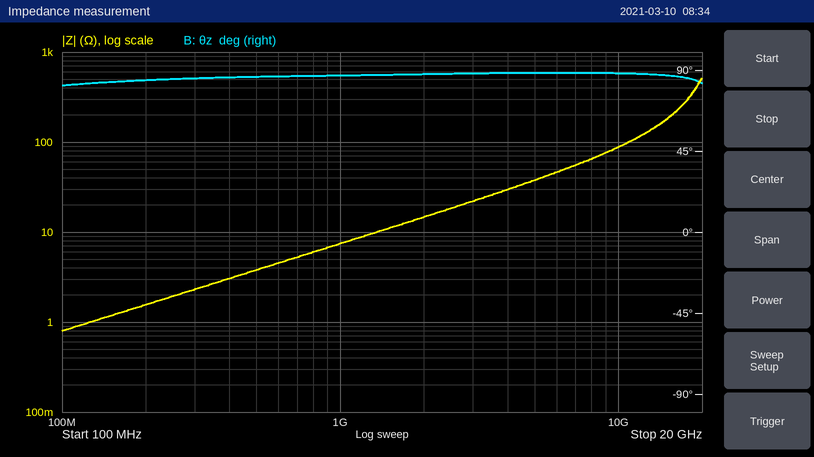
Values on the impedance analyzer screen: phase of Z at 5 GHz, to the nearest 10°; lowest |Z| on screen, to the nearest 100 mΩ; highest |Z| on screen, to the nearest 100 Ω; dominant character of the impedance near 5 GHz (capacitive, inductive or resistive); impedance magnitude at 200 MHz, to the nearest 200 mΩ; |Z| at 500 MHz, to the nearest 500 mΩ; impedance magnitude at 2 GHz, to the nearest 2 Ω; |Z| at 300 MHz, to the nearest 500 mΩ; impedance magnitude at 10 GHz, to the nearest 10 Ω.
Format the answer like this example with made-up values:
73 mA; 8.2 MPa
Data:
90°; 800 mΩ; 500 Ω; inductive; 1.6 Ω; 4.0 Ω; 14 Ω; 2.5 Ω; 90 Ω
